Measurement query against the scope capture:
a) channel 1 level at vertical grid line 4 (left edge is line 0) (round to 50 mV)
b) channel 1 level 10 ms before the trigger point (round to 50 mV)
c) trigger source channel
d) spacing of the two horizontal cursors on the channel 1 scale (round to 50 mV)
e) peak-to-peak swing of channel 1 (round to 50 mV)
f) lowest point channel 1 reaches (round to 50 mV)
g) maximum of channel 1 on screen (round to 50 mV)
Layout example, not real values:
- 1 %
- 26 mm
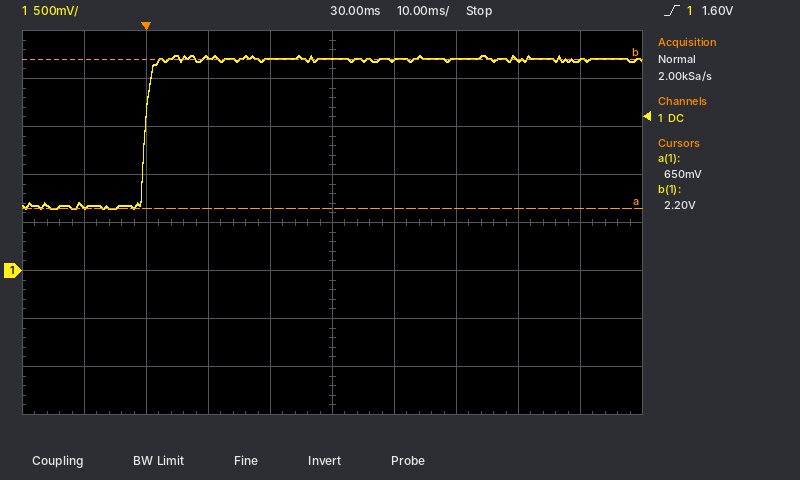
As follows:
- 2.20 V
- 650 mV
- channel 1
- 1.55 V
- 1.60 V
- 650 mV
- 2.25 V
